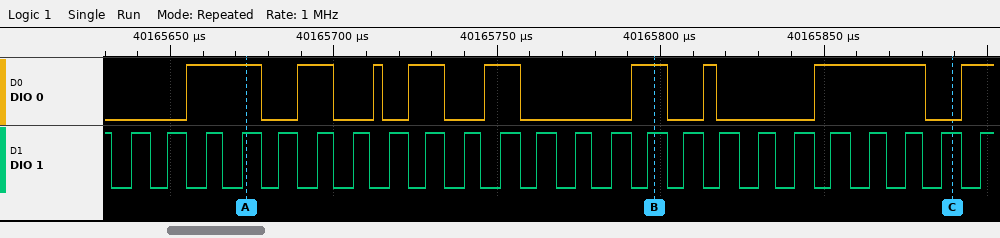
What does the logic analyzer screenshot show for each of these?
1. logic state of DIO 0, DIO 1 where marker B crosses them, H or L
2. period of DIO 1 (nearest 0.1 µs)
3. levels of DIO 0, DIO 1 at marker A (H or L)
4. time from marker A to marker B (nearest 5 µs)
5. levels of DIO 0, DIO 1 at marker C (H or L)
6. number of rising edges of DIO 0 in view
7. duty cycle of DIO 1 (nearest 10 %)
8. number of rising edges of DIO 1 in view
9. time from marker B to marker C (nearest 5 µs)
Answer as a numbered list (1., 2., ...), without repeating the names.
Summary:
1. DIO 0=H, DIO 1=H
2. 11.3 µs
3. DIO 0=H, DIO 1=H
4. 125 µs
5. DIO 0=L, DIO 1=H
6. 9
7. 50 %
8. 24
9. 90 µs
